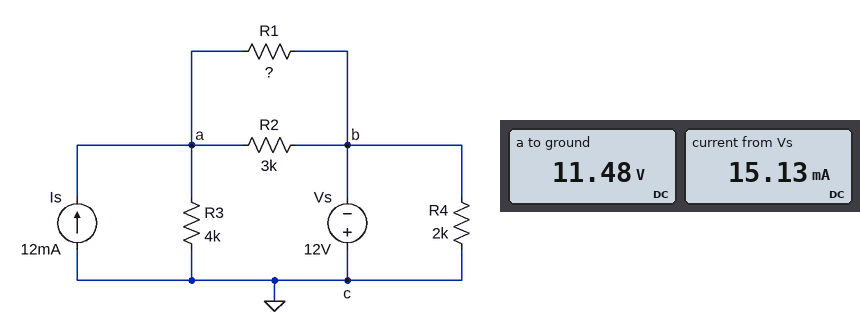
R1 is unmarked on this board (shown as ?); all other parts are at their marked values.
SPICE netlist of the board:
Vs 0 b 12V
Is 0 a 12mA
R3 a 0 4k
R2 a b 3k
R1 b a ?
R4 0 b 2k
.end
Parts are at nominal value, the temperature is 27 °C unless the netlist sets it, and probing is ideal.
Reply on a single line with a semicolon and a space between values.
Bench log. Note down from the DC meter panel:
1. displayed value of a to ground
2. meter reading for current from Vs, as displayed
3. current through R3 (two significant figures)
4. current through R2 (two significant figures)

11.48 V; 15.13 mA; 2.9 mA; 7.8 mA
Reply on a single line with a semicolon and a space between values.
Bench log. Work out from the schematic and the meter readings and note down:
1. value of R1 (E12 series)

18 kΩ
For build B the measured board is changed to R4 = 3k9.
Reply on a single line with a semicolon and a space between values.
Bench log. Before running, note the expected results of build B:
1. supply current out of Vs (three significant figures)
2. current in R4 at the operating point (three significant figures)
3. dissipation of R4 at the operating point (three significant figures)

12.2 mA; 3.08 mA; 36.9 mW
